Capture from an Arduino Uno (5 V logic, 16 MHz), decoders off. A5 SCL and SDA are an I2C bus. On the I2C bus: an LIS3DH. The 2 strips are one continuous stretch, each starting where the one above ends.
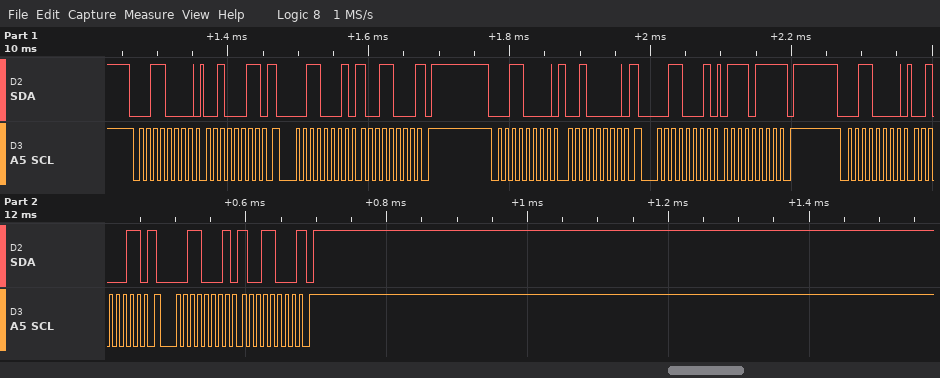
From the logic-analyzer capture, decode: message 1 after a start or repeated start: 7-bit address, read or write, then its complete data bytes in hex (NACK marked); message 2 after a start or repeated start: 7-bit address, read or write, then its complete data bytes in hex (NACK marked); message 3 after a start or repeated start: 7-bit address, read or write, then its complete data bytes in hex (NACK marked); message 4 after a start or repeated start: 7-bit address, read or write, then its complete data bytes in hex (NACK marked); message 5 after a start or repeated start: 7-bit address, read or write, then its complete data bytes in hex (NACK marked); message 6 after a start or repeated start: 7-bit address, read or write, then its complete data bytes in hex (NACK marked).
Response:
0x18 write: 23
0x18 read: 98 NACK
0x18 write: 20
0x18 read: 77 NACK
0x18 write: 23
0x18 read: 98 NACK
